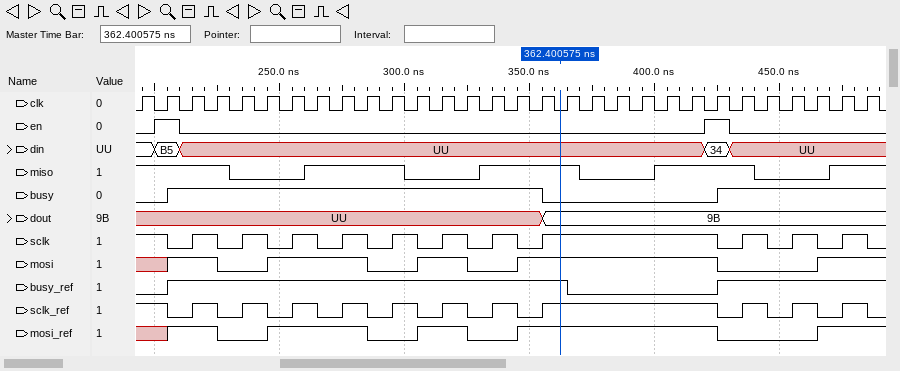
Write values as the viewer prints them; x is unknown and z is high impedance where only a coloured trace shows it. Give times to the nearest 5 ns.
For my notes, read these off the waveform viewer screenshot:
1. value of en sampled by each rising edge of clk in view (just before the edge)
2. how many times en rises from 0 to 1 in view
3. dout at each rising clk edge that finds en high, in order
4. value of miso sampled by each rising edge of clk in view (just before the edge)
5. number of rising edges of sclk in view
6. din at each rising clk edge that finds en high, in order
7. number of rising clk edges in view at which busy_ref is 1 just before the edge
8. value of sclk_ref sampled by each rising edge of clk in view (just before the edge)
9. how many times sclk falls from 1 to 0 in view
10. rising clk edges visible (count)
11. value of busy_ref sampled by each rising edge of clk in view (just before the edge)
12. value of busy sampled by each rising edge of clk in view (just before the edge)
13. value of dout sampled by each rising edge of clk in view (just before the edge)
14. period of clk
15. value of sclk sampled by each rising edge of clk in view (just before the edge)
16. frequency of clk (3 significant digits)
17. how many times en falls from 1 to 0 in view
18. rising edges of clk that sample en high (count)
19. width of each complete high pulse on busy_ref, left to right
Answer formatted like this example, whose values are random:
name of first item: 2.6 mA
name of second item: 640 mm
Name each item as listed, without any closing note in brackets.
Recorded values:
value of en sampled by each rising edge of clk in view: 0 1 0 0 0 0 0 0 0 0 0 0 0 0 0 0 0 0 0 0 0 0 0 1 0 0 0 0 0 0
how many times en rises from 0 to 1 in view: 2
dout at each rising clk edge that finds en high, in order: UU, 9B
value of miso sampled by each rising edge of clk in view: 1 1 1 1 0 0 0 1 1 1 1 0 0 0 1 1 1 1 0 0 0 1 1 1 1 0 0 0 1 1
number of rising edges of sclk in view: 11
din at each rising clk edge that finds en high, in order: B5, 34
number of rising clk edges in view at which busy_ref is 1 just before the edge: 22
value of sclk_ref sampled by each rising edge of clk in view: 1 1 0 1 0 1 0 1 0 1 0 1 0 1 0 1 0 1 1 1 1 1 1 1 0 1 0 1 0 1
how many times sclk falls from 1 to 0 in view: 12
rising clk edges visible: 30
value of busy_ref sampled by each rising edge of clk in view: 0 0 1 1 1 1 1 1 1 1 1 1 1 1 1 1 1 1 0 0 0 0 0 0 1 1 1 1 1 1
value of busy sampled by each rising edge of clk in view: 0 0 1 1 1 1 1 1 1 1 1 1 1 1 1 1 1 0 0 0 0 0 0 0 1 1 1 1 1 1
value of dout sampled by each rising edge of clk in view: UU, UU, UU, UU, UU, UU, UU, UU, UU, UU, UU, UU, UU, UU, UU, UU, UU, 9B, 9B, 9B, 9B, 9B, 9B, 9B, 9B, 9B, 9B, 9B, 9B, 9B
period of clk: 10 ns
value of sclk sampled by each rising edge of clk in view: 1 1 0 1 0 1 0 1 0 1 0 1 0 1 0 1 0 1 1 1 1 1 1 1 0 1 0 1 0 1
frequency of clk: 100 MHz
how many times en falls from 1 to 0 in view: 2
rising edges of clk that sample en high: 2
width of each complete high pulse on busy_ref, left to right: 160 ns
